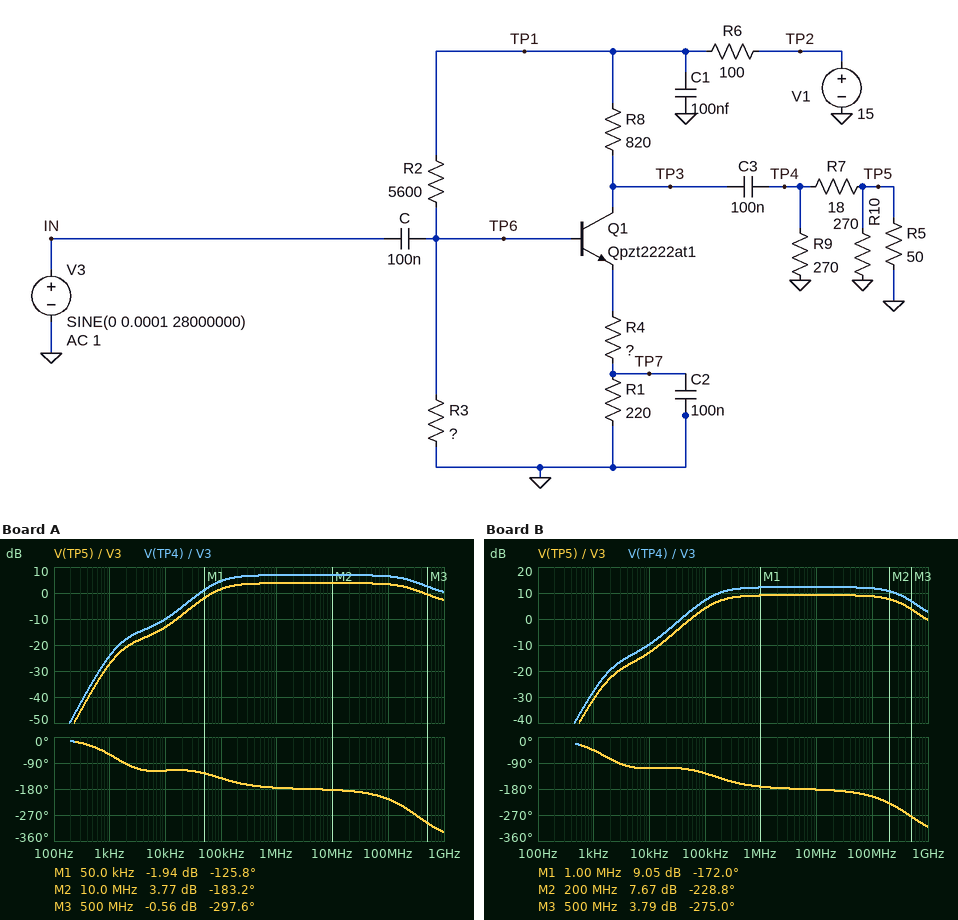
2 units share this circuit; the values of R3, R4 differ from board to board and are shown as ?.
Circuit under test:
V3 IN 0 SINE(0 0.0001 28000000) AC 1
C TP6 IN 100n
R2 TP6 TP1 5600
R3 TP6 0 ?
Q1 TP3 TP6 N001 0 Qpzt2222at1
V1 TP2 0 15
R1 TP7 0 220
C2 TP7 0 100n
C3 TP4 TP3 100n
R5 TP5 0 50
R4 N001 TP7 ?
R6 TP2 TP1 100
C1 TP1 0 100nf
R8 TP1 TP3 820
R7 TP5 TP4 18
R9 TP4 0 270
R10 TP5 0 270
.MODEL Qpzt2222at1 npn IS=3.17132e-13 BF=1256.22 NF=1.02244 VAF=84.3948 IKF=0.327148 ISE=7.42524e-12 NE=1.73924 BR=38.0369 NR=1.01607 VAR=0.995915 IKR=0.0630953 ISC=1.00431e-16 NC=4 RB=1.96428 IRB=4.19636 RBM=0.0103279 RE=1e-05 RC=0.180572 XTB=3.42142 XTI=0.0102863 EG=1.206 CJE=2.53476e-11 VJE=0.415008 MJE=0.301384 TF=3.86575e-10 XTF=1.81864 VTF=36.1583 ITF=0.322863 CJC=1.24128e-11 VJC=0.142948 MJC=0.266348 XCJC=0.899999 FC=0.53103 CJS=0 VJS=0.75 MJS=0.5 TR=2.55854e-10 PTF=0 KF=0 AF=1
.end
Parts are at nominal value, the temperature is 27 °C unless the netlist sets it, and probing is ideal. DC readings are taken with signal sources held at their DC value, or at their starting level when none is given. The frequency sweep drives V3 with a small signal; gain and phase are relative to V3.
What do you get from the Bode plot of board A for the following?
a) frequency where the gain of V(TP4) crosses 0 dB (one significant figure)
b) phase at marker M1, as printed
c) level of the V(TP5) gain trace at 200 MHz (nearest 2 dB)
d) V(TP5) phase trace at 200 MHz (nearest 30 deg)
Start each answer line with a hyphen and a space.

- 40 kHz
- -125.8 deg
- 2 dB
- -240 deg
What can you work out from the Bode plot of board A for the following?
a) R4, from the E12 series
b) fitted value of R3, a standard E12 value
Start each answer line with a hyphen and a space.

- 18 Ω
- 1.8 kΩ
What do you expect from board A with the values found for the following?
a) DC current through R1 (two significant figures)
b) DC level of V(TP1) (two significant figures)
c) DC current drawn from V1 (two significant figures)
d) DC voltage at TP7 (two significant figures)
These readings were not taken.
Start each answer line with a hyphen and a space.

- 11 mA
- 14 V
- 13 mA
- 2.4 V
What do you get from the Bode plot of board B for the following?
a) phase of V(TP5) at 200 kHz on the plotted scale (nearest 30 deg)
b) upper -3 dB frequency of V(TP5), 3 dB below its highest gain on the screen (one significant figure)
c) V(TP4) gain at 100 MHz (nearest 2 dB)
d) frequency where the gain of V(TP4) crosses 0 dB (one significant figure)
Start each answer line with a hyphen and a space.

- -150 deg
- 300 MHz
- 12 dB
- 40 kHz
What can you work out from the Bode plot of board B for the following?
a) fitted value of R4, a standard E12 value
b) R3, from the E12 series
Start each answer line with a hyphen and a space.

- 5.6 Ω
- 820 Ω
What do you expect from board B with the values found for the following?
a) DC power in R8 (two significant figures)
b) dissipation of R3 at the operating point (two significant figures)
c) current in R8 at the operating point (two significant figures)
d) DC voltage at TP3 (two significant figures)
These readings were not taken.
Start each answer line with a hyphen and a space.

- 22 mW
- 4.0 mW
- 5.1 mA
- 10 V
